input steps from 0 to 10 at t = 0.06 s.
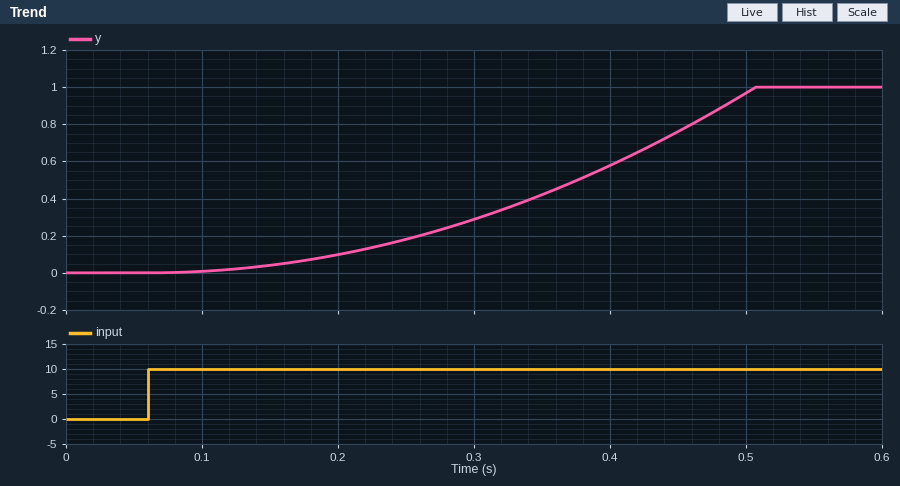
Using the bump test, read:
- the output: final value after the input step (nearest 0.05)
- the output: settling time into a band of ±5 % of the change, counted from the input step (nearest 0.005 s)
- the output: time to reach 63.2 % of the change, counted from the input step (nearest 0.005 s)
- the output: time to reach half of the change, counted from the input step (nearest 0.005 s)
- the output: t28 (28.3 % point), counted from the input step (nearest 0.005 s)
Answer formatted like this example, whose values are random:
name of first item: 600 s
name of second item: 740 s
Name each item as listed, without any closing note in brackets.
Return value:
the output: final value after the input step: 1.00
the output: settling time into a band of ±5 % of the change, counted from the input step: 0.435 s
the output: time to reach 63.2 % of the change, counted from the input step: 0.355 s
the output: time to reach half of the change, counted from the input step: 0.315 s
the output: t28 (28.3 % point), counted from the input step: 0.240 s
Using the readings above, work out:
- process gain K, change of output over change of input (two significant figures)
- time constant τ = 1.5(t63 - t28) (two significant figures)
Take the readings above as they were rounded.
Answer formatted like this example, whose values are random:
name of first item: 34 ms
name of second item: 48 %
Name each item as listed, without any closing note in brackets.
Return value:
process gain K, change of output over change of input: 0.10
time constant τ = 1.5(t63 - t28): 0.17 s
